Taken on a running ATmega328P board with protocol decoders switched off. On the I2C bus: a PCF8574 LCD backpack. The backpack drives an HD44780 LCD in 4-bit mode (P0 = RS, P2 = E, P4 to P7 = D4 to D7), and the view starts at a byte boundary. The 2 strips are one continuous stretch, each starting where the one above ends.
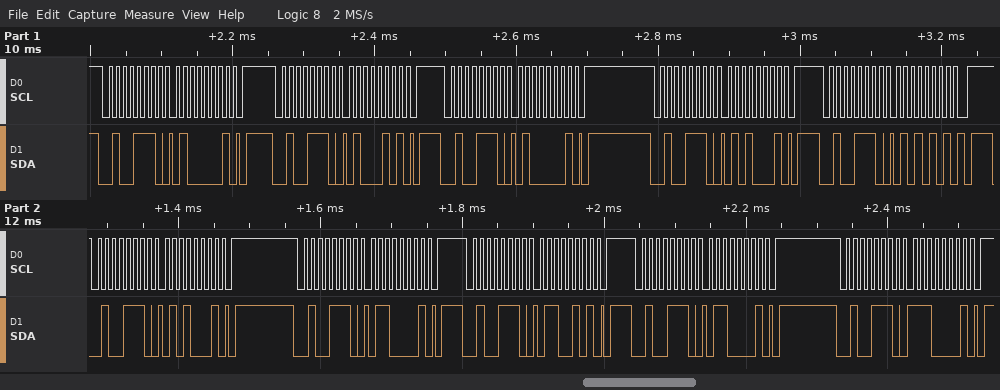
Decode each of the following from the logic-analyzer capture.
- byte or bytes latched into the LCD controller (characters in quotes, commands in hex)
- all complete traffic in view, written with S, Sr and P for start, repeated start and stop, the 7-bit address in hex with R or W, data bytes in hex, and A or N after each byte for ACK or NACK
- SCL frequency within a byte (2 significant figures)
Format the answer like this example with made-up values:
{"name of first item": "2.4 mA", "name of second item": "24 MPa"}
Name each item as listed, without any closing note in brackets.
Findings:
{"byte or bytes latched into the LCD controller": "'E'", "all complete traffic in view, written with S, Sr and P for start, repeated start and stop, the 7-bit address in hex with R or W, data bytes in hex, and A or N after each byte for ACK or NACK": "S 27W A 41 A P S 27W A 45 A P S 27W A 41 A P S 27W A 51 A P S 27W A 55 A P S 27W A 51 A P S 27W A 61 A P S 27W A 65 A P S 27W A 61 A P S 27W A E1 A P", "SCL frequency within a byte": "100 kHz"}
